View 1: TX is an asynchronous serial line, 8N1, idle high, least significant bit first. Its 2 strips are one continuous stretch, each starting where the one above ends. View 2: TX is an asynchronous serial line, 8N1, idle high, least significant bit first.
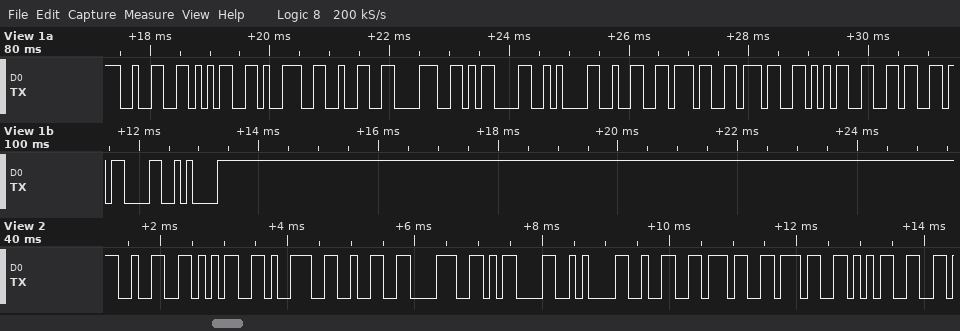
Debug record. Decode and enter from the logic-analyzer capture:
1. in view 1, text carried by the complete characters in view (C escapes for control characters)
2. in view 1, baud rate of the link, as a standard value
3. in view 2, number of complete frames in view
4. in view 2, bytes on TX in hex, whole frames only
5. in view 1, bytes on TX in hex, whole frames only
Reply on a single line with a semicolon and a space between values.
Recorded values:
"25928\r\n27756\r\n"; 9600 baud; 11; 0x32 0x35 0x39 0x32 0x38 0x0D 0x0A 0x32 0x37 0x37 0x35; 32 35 39 32 38 0D 0A 32 37 37 35 36 0D 0A
